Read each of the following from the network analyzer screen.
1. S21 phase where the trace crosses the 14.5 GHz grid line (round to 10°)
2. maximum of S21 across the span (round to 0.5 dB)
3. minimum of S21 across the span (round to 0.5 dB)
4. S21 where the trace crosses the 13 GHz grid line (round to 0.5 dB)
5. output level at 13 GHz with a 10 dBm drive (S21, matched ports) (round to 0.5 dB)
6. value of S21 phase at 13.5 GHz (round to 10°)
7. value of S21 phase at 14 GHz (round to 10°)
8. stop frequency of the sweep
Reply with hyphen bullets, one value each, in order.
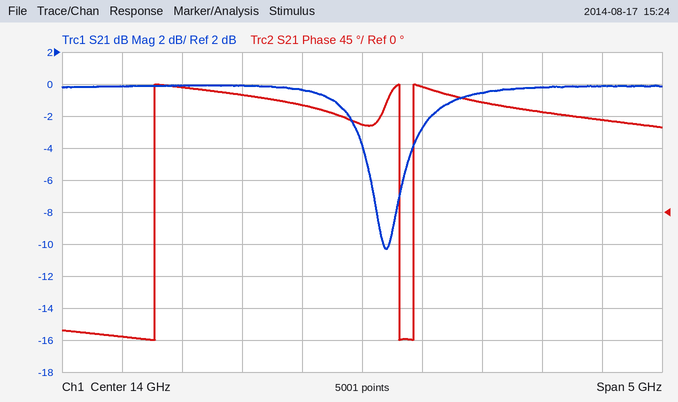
- 180°
- 0.0 dB
- -10.5 dB
- 0.0 dB
- 10.0 dBm
- 150°
- 120°
- 16.5 GHz
